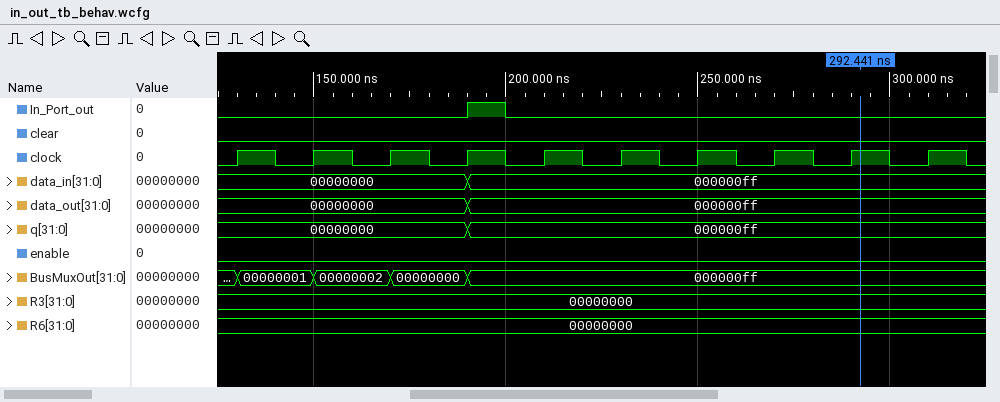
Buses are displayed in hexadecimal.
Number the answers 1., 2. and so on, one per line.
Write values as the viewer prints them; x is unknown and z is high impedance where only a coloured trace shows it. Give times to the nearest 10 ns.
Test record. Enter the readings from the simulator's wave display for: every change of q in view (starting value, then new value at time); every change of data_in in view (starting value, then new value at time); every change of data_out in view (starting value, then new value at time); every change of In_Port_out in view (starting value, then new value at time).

1. 00000000, 000000ff at 190 ns
2. 00000000, 000000ff at 190 ns
3. 00000000, 000000ff at 190 ns
4. 0, 1 at 190 ns, 0 at 200 ns
